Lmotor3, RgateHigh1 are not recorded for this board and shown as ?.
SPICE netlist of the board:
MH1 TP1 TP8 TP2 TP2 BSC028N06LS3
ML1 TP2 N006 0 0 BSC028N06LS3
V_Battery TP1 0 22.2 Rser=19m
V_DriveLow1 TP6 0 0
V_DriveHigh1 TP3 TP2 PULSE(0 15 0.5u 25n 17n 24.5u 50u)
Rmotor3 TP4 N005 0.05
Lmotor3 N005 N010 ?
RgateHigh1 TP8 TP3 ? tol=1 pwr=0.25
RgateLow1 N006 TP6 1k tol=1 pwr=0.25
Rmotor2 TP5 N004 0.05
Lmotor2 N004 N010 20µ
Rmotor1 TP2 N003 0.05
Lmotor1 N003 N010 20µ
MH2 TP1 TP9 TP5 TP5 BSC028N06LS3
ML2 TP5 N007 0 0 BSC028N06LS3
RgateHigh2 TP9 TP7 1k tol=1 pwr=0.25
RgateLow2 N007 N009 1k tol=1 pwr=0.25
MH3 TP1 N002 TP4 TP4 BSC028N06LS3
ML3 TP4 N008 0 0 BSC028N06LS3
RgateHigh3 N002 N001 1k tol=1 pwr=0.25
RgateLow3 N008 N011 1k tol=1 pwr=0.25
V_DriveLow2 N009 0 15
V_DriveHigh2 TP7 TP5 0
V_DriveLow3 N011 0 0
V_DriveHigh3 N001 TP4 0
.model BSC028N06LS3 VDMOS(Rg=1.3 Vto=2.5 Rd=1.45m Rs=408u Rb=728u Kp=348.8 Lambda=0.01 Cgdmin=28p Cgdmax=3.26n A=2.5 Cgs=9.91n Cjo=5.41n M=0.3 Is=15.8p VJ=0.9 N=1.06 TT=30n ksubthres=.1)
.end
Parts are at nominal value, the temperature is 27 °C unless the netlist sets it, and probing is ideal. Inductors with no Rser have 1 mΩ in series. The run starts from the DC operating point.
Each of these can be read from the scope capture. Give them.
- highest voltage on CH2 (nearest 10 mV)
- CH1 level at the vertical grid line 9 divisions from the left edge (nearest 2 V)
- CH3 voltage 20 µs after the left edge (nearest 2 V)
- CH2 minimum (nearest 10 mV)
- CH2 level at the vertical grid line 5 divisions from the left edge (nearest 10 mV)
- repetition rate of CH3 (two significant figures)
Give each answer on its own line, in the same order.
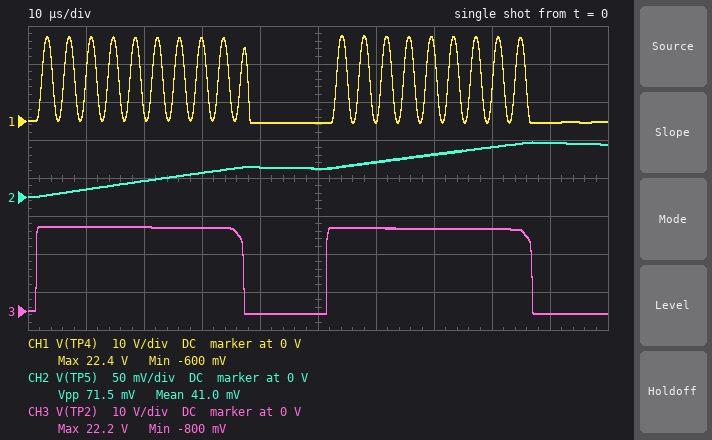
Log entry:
70 mV
0 V
22 V
0 V
40 mV
20 kHz
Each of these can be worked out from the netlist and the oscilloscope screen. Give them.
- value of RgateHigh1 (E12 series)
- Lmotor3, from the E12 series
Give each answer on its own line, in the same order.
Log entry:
470 Ω
56 µH
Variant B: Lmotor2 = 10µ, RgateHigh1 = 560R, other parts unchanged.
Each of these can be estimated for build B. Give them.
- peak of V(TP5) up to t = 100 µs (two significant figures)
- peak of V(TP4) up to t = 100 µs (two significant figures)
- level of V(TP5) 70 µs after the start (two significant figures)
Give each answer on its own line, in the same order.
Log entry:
96 mV
17 V
74 mV
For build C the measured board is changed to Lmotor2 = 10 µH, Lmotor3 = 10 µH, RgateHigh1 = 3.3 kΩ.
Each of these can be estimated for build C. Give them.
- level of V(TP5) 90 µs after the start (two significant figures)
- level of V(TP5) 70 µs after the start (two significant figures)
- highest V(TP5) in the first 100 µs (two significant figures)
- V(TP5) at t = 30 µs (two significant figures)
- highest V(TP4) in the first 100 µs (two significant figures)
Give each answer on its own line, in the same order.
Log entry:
110 mV
86 mV
120 mV
34 mV
13 V
